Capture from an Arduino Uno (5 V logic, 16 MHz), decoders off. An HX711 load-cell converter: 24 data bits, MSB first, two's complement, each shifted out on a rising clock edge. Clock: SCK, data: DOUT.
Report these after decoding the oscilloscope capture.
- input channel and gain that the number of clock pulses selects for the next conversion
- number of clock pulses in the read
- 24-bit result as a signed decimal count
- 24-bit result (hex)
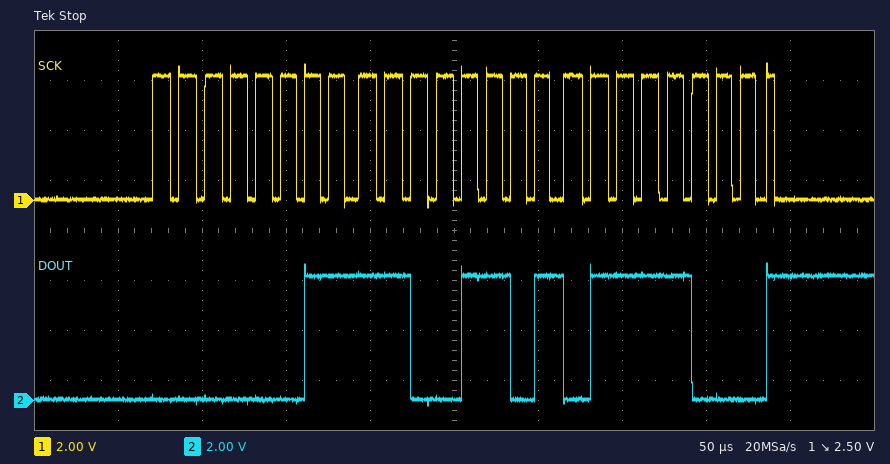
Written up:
channel A, gain 128
25
249208
0x03CD78
